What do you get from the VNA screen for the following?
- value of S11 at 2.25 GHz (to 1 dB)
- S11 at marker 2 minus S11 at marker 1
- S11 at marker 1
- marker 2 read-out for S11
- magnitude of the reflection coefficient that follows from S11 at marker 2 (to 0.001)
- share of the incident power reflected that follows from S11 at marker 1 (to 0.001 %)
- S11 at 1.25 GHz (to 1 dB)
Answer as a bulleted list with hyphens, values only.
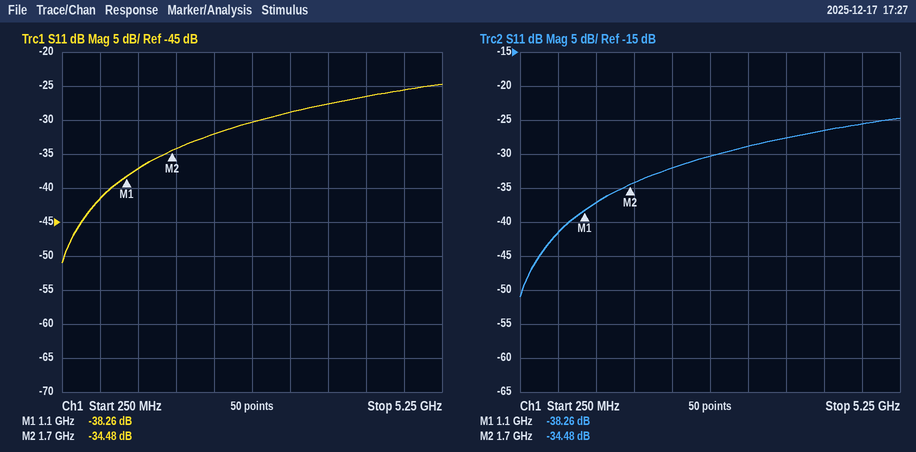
- -32 dB
- 3.78 dB
- -38.26 dB
- -34.48 dB
- 0.019
- 0.015 %
- -37 dB
